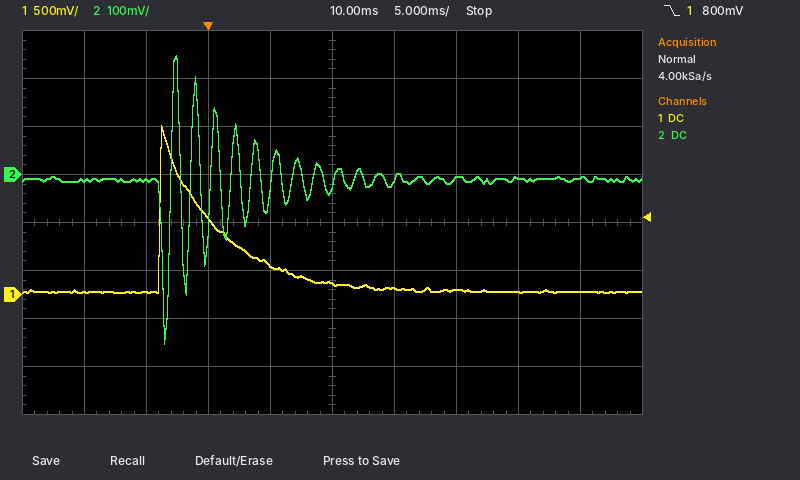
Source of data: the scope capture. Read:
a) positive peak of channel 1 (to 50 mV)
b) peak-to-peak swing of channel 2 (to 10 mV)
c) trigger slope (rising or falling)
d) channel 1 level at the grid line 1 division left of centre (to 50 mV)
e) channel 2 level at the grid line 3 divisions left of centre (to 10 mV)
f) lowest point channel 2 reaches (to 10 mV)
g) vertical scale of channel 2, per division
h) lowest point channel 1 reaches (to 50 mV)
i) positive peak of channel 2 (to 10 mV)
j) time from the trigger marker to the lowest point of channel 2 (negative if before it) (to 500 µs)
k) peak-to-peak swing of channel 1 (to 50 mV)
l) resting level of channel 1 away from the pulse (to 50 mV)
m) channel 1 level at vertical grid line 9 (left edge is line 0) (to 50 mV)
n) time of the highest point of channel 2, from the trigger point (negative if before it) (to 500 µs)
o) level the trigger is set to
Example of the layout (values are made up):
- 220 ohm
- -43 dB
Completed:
- 1.75 V
- 600 mV
- falling
- 300 mV
- -10 mV
- -350 mV
- 100 mV
- 0 mV
- 250 mV
- -3.5 ms
- 1.75 V
- 50 mV
- 50 mV
- -2.5 ms
- 800 mV
